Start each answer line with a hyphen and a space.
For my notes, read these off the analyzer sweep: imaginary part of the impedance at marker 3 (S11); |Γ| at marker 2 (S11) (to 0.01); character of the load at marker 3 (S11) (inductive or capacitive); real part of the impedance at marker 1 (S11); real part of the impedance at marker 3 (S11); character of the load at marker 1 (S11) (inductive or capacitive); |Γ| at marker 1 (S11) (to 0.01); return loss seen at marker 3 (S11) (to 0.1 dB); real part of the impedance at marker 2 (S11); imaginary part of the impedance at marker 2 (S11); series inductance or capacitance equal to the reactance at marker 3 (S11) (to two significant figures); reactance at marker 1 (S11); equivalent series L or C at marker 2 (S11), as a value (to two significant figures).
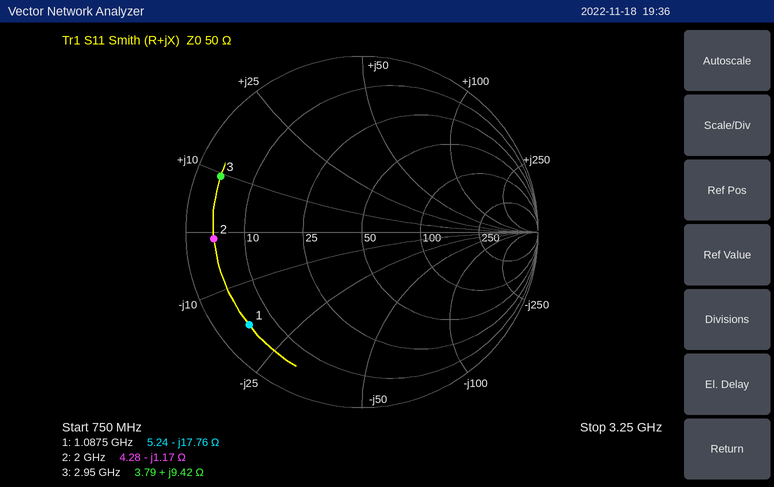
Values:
- +9.42 Ω
- 0.84
- inductive
- 5.24 Ω
- 3.79 Ω
- capacitive
- 0.83
- 1.3 dB
- 4.28 Ω
- -1.17 Ω
- 510 pH
- -17.76 Ω
- 68 pF
